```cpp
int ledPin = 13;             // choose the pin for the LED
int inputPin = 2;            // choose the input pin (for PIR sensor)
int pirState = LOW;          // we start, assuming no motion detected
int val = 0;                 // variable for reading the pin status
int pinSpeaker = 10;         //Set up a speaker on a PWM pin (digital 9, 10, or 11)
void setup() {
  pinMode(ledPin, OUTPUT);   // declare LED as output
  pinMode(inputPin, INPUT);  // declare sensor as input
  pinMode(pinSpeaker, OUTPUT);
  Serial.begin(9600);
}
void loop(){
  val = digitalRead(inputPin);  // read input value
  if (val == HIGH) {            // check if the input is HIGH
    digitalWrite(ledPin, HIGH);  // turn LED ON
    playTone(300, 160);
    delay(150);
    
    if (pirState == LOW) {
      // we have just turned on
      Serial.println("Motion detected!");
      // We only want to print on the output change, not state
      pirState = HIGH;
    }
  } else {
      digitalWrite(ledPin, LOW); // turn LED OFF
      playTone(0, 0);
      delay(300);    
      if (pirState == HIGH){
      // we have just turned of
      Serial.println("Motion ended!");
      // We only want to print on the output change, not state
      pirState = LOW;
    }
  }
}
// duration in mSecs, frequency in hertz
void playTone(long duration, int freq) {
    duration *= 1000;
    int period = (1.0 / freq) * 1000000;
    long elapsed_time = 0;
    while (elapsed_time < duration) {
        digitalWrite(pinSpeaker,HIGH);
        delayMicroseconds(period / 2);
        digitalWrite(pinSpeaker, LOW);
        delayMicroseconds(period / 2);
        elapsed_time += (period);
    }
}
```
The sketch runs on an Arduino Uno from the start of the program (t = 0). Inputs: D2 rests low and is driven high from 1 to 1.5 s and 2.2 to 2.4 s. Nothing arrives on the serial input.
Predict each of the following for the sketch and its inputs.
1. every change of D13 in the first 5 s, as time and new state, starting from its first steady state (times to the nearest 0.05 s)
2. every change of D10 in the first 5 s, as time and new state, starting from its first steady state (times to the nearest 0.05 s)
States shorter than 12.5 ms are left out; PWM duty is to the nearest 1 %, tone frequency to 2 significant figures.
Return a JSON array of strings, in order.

["0 s low; 1.2 s high; 1.65 s low; 2.25 s high; 2.7 s low", "0 s low; 1.2 s tone 160 Hz; 1.5 s low; 2.25 s tone 160 Hz; 2.55 s low"]
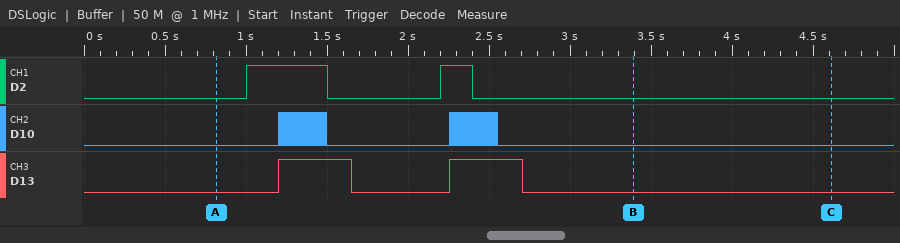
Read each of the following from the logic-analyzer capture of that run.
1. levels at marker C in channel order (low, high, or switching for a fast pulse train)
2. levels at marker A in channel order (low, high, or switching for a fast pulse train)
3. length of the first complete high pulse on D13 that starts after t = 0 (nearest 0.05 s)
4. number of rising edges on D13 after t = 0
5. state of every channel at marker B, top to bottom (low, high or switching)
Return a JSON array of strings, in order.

["D2 low, D10 low, D13 low", "D2 low, D10 low, D13 low", "0.45 s", "2", "D2 low, D10 low, D13 low"]
